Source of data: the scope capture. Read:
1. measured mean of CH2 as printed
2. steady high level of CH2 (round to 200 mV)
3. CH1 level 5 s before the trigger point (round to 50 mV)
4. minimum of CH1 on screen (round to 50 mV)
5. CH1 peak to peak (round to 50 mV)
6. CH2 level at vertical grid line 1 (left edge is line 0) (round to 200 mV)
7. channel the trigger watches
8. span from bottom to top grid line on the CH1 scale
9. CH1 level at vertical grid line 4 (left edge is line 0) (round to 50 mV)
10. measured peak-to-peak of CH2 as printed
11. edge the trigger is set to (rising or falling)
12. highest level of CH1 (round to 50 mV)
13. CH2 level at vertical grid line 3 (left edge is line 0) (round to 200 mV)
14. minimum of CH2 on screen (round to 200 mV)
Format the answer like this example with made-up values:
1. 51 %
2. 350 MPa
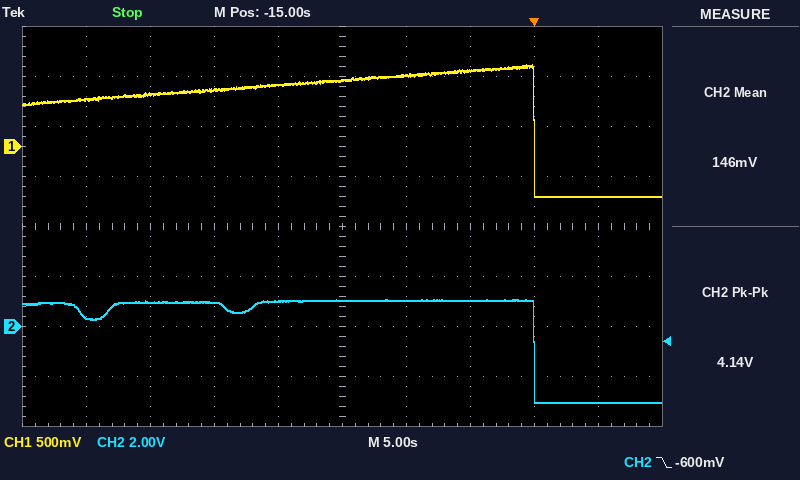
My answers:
1. 146 mV
2. 1.0 V
3. 750 mV
4. -500 mV
5. 1.30 V
6. 400 mV
7. CH2
8. 4 V
9. 600 mV
10. 4.14 V
11. falling
12. 800 mV
13. 1.0 V
14. -3.0 V
